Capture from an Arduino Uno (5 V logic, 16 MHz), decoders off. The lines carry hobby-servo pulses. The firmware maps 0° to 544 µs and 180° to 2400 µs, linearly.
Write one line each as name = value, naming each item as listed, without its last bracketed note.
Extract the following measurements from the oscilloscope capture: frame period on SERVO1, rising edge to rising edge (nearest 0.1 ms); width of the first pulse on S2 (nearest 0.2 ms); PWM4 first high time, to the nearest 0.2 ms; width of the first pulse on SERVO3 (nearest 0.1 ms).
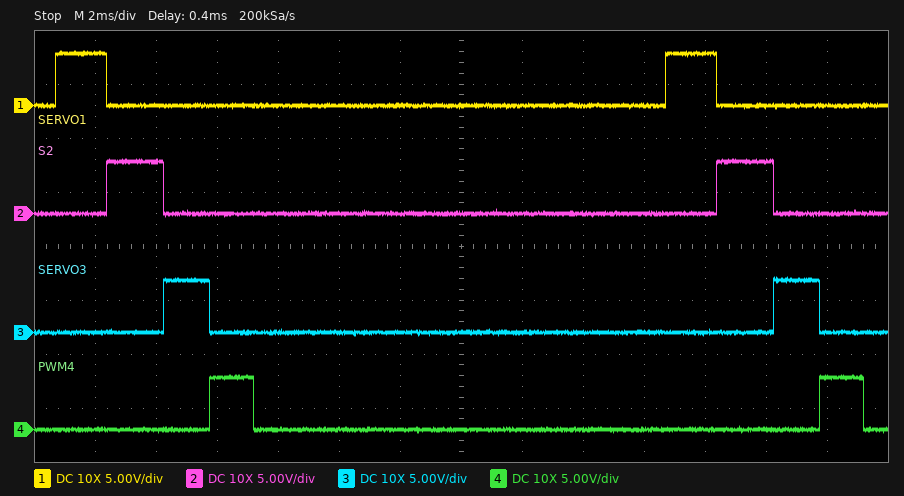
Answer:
frame period on SERVO1, rising edge to rising edge = 20.0 ms
width of the first pulse on S2 = 1.8 ms
PWM4 first high time, to the nearest 0.2 ms = 1.4 ms
width of the first pulse on SERVO3 = 1.5 ms
